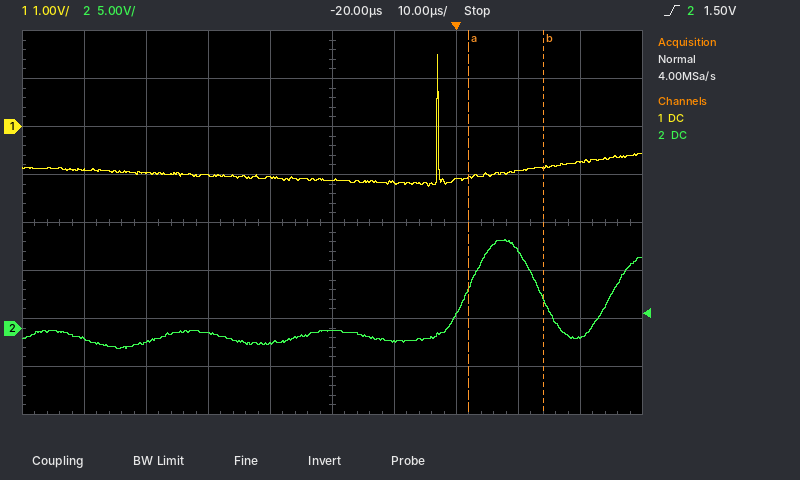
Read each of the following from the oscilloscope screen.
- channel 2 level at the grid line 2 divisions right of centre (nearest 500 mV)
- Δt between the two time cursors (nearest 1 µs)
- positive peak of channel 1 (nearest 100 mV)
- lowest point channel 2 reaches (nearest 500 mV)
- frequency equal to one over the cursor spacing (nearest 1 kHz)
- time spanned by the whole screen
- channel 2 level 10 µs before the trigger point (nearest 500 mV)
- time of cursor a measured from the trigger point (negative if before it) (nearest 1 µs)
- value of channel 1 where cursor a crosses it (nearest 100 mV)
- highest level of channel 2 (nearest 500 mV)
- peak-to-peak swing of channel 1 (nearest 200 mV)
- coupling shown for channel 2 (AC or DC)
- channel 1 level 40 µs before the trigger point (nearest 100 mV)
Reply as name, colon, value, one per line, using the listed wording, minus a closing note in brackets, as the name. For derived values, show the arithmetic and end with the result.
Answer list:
channel 2 level at the grid line 2 divisions right of centre: 1.5 V
Δt between the two time cursors: 12 µs
positive peak of channel 1: 1.5 V
lowest point channel 2 reaches: -2.0 V
frequency equal to one over the cursor spacing: 1 / 12 µs ≈ 83 kHz
time spanned by the whole screen: 100 µs
channel 2 level 10 µs before the trigger point: -1.5 V
time of cursor a measured from the trigger point (negative if before it): +2 µs
value of channel 1 where cursor a crosses it: -1.1 V
highest level of channel 2: 9.0 V
peak-to-peak swing of channel 1: 2.8 V
coupling shown for channel 2: DC
channel 1 level 40 µs before the trigger point: -1.0 V
